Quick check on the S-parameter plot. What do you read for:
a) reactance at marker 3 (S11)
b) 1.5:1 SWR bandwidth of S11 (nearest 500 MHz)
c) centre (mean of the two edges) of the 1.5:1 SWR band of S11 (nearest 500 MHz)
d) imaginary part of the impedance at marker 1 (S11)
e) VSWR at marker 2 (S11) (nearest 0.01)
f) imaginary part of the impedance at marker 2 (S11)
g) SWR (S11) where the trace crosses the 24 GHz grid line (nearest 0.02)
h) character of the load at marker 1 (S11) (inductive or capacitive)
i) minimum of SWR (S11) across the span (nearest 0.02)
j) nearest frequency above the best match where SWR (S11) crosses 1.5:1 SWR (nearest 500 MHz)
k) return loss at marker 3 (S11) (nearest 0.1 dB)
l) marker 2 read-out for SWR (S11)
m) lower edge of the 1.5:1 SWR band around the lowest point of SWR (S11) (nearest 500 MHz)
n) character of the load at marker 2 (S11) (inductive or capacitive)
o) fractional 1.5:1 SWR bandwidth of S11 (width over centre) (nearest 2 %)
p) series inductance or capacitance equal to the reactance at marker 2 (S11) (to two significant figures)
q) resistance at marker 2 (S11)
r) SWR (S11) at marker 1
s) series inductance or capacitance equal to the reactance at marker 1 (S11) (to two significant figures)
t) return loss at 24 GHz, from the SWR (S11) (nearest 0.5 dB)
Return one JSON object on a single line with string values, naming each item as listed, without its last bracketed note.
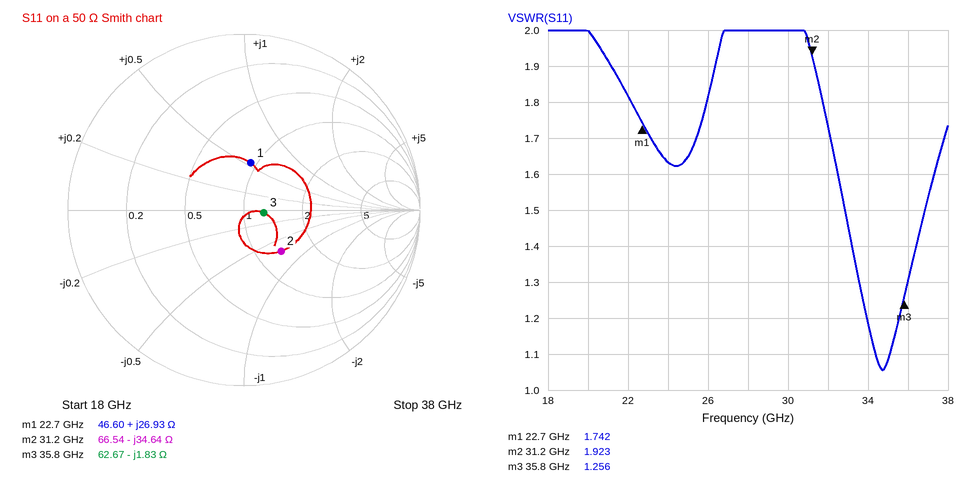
{"reactance at marker 3": "-1.83 Ω", "1.5:1 SWR bandwidth of S11": "4.0 GHz", "centre (mean of the two edges) of the 1.5:1 SWR band of S11": "35.0 GHz", "imaginary part of the impedance at marker 1": "+26.93 Ω", "VSWR at marker 2 (S11)": "1.92", "imaginary part of the impedance at marker 2": "-34.64 Ω", "SWR (S11) where the trace crosses the 24 GHz grid line": "1.64", "character of the load at marker 1 (S11)": "inductive", "minimum of SWR (S11) across the span": "1.06", "nearest frequency above the best match where SWR (S11) crosses 1.5:1 SWR": "37.0 GHz", "return loss at marker 3 (S11)": "18.9 dB", "marker 2 read-out for SWR": "1.923", "lower edge of the 1.5:1 SWR band around the lowest point of SWR (S11)": "33.0 GHz", "character of the load at marker 2 (S11)": "capacitive", "fractional 1.5:1 SWR bandwidth of S11 (width over centre)": "12 %", "series inductance or capacitance equal to the reactance at marker 2 (S11)": "150 fF", "resistance at marker 2": "66.54 Ω", "SWR (S11) at marker 1": "1.742", "series inductance or capacitance equal to the reactance at marker 1 (S11)": "190 pH", "return loss at 24 GHz, from the SWR (S11)": "12.5 dB"}
